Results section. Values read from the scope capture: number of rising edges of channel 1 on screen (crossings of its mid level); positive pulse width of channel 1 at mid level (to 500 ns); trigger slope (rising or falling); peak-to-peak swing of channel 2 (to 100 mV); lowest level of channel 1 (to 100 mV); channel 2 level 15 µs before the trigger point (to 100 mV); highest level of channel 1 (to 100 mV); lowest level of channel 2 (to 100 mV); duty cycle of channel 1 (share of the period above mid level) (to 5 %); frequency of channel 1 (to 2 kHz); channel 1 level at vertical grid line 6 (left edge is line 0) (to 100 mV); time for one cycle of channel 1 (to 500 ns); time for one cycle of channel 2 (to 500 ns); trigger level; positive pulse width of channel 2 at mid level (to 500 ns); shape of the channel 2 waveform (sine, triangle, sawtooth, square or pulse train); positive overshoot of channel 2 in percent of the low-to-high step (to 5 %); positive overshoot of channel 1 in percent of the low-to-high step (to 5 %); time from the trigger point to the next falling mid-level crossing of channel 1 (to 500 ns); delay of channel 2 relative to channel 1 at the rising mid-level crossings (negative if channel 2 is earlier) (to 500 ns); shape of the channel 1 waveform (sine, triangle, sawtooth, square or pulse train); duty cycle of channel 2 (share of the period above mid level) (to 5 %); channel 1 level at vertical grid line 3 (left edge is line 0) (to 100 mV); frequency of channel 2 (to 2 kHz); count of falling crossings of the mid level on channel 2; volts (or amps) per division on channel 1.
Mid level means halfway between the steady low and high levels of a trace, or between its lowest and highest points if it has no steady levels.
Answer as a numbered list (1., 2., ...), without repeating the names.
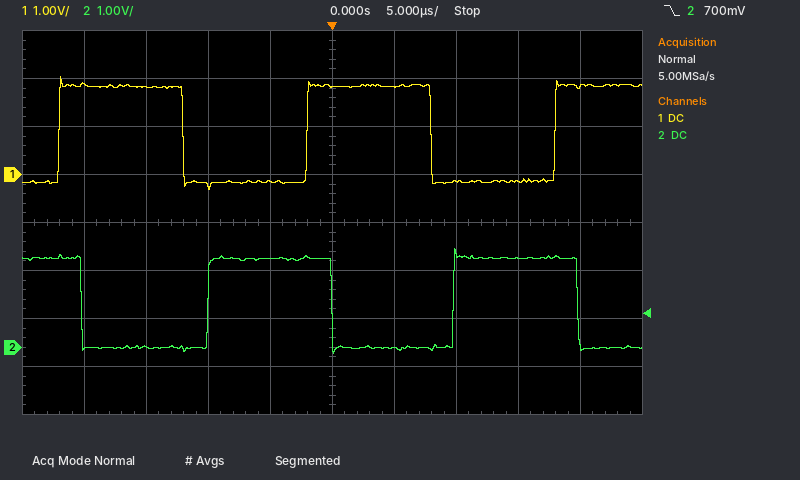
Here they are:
1. 3
2. 10.0 µs
3. falling
4. 2.2 V
5. -300 mV
6. 0.0 V
7. 2.0 V
8. -100 mV
9. 50 %
10. 50 kHz
11. 1.8 V
12. 20.0 µs
13. 20.0 µs
14. 700 mV
15. 10.0 µs
16. square
17. 10 %
18. 10 %
19. 8.0 µs
20. -8.0 µs
21. square
22. 50 %
23. -200 mV
24. 50 kHz
25. 3
26. 1 V
